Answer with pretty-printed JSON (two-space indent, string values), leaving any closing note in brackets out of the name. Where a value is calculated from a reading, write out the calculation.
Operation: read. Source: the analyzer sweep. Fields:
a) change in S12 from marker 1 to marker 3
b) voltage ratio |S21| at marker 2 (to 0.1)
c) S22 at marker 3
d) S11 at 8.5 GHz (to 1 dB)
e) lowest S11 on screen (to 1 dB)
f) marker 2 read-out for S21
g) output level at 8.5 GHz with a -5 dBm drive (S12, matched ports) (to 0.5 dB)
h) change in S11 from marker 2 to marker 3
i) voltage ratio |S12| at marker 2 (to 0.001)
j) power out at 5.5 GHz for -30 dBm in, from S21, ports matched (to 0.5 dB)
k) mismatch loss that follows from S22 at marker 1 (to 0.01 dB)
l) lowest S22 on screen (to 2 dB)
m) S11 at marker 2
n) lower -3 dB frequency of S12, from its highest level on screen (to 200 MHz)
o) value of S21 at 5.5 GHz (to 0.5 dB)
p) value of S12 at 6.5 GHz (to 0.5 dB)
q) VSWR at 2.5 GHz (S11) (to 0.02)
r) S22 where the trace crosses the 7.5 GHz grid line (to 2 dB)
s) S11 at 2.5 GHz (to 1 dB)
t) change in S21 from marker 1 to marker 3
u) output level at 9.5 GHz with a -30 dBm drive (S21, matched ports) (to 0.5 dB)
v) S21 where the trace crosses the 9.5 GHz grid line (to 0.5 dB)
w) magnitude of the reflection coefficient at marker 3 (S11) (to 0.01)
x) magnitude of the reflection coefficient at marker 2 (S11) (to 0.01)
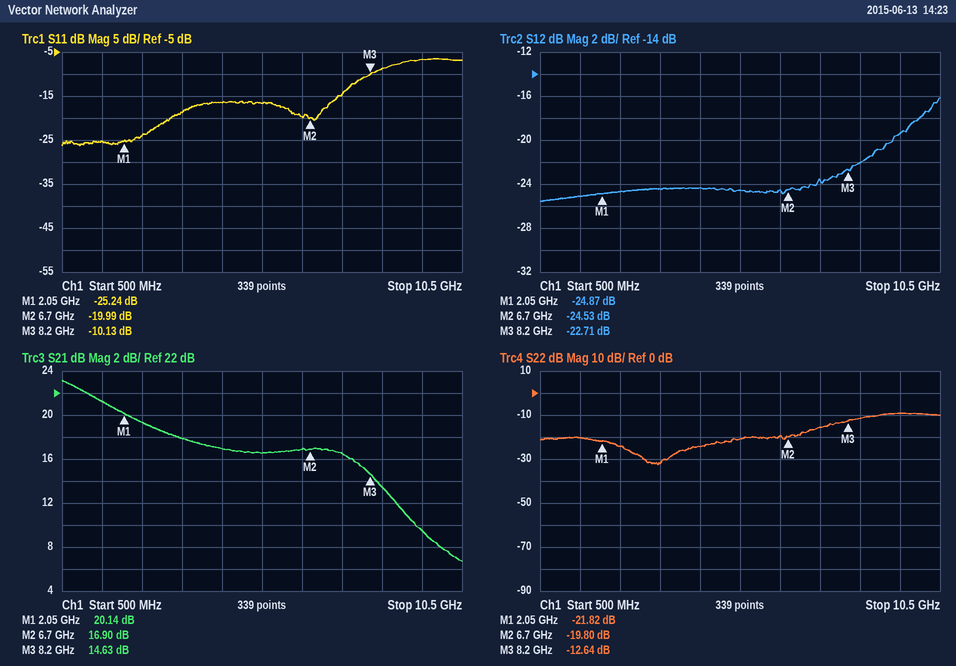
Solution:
{
  "change in S12 from marker 1 to marker 3": "-22.71 − (-24.87) = 2.16 dB",
  "voltage ratio |S21| at marker 2": "10^(16.9/20) ≈ 7.0",
  "S22 at marker 3": "-12.64 dB",
  "S11 at 8.5 GHz": "-9 dB",
  "lowest S11 on screen": "-26 dB",
  "marker 2 read-out for S21": "16.90 dB",
  "output level at 8.5 GHz with a -5 dBm drive (S12, matched ports)": "-5 dBm + (-22.0 dB) = -27.0 dBm",
  "change in S11 from marker 2 to marker 3": "-10.13 − (-19.99) = 9.86 dB",
  "voltage ratio |S12| at marker 2": "10^(-24.53/20) ≈ 0.059",
  "power out at 5.5 GHz for -30 dBm in, from S21, ports matched": "-30 dBm + (16.5 dB) = -13.5 dBm",
  "mismatch loss that follows from S22 at marker 1": "−10 log10(1 − 10^(-21.82/10)) ≈ 0.03 dB",
  "lowest S22 on screen": "-32 dB",
  "S11 at marker 2": "-19.99 dB",
  "lower -3 dB frequency of S12, from its highest level on screen": "9.6 GHz",
  "value of S21 at 5.5 GHz": "16.5 dB",
  "value of S12 at 6.5 GHz": "-24.5 dB",
  "VSWR at 2.5 GHz (S11)": "|Γ| = 10^(-24/20) = 0.0631; VSWR = (1 + 0.0631)/(1 − 0.0631) ≈ 1.13, so 1.14 to the nearest 0.02",
  "S22 where the trace crosses the 7.5 GHz grid line": "-16 dB",
  "S11 at 2.5 GHz": "-24 dB",
  "change in S21 from marker 1 to marker 3": "14.63 − (20.14) = -5.51 dB",
  "output level at 9.5 GHz with a -30 dBm drive (S21, matched ports)": "-30 dBm + (9.5 dB) = -20.5 dBm",
  "S21 where the trace crosses the 9.5 GHz grid line": "9.5 dB",
  "magnitude of the reflection coefficient at marker 3 (S11)": "10^(-10.13/20) ≈ 0.31",
  "magnitude of the reflection coefficient at marker 2 (S11)": "10^(-19.99/20) ≈ 0.10"
}
